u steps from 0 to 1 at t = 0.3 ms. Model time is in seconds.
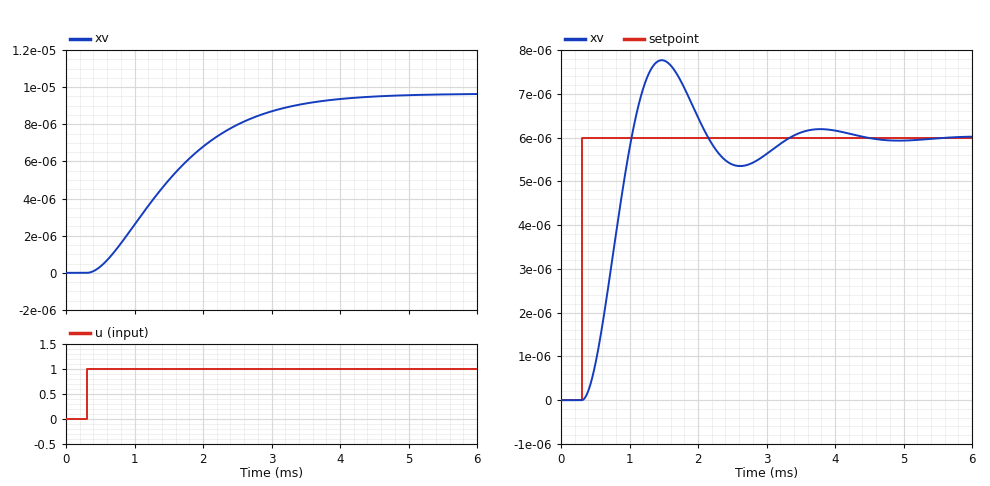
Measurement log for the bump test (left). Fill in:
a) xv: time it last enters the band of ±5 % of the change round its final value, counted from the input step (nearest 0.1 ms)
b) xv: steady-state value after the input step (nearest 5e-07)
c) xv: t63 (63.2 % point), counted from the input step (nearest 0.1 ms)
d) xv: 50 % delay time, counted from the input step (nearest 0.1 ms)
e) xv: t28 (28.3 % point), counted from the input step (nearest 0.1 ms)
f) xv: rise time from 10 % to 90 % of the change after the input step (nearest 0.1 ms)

3.3 ms
0.0000095
1.5 ms
1.2 ms
0.7 ms
2.3 ms
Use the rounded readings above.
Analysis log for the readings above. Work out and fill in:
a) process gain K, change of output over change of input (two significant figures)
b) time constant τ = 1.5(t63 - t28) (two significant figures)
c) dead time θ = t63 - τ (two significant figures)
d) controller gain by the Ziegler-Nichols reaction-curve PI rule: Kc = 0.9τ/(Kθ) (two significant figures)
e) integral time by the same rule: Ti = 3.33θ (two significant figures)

0.0000095
1.2 ms
0.30 ms
380000
1.00 ms
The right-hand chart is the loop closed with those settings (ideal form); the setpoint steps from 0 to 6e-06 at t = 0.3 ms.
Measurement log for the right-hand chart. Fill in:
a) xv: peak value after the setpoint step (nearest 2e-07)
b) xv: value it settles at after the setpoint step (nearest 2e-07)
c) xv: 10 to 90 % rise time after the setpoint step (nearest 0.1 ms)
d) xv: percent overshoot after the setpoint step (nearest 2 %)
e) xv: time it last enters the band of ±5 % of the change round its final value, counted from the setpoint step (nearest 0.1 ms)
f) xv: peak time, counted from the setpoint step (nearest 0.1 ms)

0.0000078
0.0000060
0.5 ms
30 %
2.8 ms
1.2 ms
